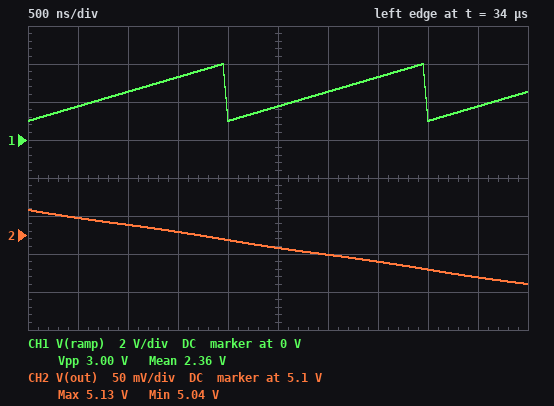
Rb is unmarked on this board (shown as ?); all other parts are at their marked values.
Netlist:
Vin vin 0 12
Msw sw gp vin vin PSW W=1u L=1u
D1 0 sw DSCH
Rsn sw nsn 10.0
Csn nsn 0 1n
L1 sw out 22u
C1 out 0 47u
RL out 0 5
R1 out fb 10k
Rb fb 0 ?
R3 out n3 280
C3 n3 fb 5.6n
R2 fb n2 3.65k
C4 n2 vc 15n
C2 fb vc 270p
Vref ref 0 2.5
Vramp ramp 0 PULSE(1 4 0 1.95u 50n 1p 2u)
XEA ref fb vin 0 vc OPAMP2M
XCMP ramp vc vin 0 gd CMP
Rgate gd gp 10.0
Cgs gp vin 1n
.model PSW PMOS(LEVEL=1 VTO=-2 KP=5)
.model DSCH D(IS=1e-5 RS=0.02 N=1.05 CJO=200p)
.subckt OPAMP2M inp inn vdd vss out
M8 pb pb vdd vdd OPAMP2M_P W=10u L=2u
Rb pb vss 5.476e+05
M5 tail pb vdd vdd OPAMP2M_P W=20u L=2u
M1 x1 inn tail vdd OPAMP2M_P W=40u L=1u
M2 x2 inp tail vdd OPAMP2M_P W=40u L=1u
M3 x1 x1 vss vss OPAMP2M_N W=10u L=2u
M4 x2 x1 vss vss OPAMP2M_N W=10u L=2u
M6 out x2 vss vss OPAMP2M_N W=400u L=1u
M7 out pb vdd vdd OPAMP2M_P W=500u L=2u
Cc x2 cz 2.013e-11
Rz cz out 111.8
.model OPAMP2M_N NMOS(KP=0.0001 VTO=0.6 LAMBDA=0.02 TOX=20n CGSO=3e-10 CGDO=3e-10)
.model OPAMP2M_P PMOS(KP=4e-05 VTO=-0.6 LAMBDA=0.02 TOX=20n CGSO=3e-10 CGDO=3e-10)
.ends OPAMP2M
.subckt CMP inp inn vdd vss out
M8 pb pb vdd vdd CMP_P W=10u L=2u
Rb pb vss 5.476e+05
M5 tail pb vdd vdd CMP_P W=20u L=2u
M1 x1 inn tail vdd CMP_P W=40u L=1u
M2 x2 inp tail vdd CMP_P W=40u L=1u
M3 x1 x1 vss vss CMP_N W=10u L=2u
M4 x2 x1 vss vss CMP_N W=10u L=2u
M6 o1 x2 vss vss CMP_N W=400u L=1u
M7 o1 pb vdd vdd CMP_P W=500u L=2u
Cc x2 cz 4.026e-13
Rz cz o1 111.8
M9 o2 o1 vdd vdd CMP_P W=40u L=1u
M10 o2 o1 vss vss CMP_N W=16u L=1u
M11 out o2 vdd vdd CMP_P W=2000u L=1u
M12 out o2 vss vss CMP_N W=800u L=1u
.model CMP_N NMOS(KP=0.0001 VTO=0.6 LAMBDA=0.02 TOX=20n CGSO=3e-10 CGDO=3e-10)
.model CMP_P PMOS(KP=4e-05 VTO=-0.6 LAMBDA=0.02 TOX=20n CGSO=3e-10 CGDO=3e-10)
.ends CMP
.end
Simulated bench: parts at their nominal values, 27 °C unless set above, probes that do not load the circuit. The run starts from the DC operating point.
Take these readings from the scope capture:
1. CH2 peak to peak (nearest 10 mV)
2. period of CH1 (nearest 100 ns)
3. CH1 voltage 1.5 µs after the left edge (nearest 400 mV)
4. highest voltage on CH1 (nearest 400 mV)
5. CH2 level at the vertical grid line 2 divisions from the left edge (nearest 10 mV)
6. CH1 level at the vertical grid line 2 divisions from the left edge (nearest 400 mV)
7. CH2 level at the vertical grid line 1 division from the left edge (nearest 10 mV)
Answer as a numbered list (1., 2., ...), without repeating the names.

1. 100 mV
2. 2.0 µs
3. 3.2 V
4. 4.0 V
5. 5.11 V
6. 2.4 V
7. 5.12 V
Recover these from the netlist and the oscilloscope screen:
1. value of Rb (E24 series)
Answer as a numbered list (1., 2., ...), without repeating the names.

1. 7.5 kΩ
